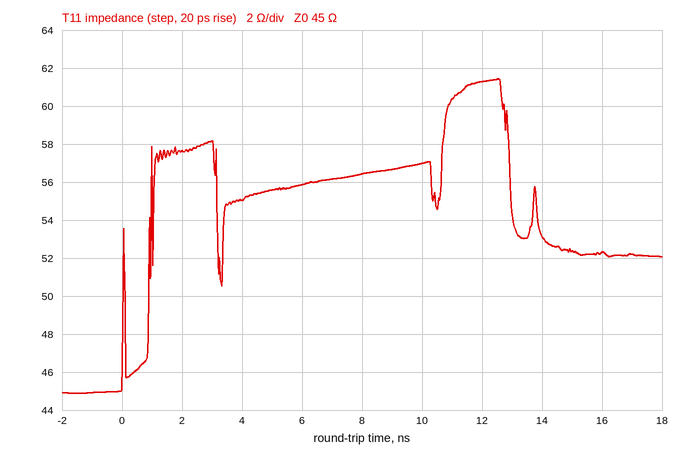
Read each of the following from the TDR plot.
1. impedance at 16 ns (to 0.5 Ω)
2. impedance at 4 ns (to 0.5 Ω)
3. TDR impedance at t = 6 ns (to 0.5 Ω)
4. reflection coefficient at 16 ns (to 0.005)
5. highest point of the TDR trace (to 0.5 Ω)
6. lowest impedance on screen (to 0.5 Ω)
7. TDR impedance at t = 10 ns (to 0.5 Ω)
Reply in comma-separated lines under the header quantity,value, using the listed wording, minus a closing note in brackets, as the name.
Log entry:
quantity,value
impedance at 16 ns,52.5 Ω
impedance at 4 ns,55.0 Ω
TDR impedance at t = 6 ns,56.0 Ω
reflection coefficient at 16 ns,+0.075
highest point of the TDR trace,61.5 Ω
lowest impedance on screen,45.0 Ω
TDR impedance at t = 10 ns,57.0 Ω
